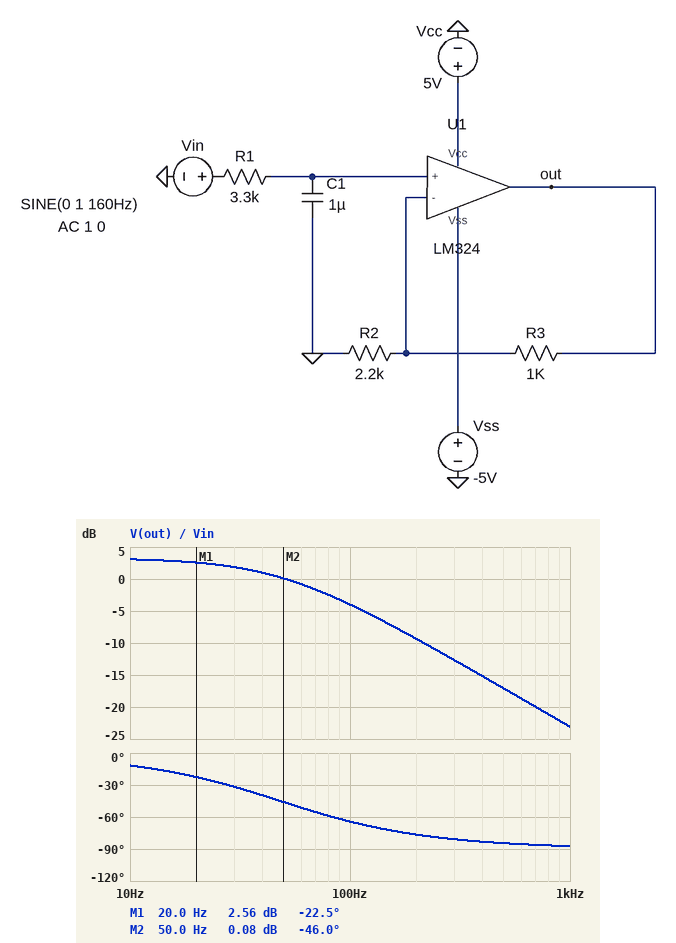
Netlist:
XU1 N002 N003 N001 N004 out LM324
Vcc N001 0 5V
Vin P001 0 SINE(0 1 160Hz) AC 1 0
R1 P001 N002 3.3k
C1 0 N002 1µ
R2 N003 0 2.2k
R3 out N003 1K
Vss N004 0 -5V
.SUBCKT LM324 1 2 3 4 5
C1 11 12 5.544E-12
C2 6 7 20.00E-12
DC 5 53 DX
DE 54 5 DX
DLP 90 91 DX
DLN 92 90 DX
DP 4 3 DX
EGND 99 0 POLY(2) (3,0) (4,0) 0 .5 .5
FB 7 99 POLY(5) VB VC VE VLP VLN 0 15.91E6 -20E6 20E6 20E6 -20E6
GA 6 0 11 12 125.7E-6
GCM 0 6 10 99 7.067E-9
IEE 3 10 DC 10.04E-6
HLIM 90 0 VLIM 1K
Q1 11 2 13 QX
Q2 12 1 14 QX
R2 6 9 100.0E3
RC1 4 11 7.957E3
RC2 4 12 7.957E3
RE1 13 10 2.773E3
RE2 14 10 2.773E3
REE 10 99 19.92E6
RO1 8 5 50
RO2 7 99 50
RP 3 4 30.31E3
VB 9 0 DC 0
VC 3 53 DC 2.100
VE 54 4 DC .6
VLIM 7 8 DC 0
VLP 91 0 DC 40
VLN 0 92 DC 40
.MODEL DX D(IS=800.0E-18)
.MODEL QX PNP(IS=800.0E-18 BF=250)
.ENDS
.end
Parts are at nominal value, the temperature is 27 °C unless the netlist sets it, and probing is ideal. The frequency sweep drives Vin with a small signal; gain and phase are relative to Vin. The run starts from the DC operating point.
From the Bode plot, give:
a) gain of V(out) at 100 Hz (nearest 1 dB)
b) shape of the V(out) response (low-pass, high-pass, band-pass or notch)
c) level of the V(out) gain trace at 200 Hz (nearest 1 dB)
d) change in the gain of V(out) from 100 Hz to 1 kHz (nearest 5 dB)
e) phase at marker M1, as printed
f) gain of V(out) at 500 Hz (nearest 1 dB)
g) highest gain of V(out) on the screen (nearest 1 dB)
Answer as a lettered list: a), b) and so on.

a) -4 dB
b) low-pass
c) -9 dB
d) -20 dB
e) -22.5 deg
f) -17 dB
g) 3 dB
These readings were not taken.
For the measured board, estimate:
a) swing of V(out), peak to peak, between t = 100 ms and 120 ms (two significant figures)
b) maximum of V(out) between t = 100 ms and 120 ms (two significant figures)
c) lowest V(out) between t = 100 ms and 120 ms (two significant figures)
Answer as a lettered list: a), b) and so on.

a) 840 mV
b) 420 mV
c) -420 mV
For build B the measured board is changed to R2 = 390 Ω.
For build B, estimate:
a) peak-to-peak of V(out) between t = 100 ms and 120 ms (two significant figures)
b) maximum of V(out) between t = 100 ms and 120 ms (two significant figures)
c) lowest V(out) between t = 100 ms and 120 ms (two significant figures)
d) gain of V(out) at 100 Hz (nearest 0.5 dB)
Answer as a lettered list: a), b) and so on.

a) 2.1 V
b) 1.0 V
c) -1.0 V
d) 4.0 dB
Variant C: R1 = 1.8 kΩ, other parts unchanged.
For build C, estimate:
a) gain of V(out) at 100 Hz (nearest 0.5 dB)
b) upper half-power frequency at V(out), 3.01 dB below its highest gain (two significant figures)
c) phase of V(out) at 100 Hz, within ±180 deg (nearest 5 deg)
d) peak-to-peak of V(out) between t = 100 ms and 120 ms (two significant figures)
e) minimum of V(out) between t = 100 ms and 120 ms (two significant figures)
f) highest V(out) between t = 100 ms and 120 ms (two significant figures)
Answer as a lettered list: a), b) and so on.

a) -0.5 dB
b) 88 Hz
c) -50 deg
d) 1.4 V
e) -700 mV
f) 700 mV
